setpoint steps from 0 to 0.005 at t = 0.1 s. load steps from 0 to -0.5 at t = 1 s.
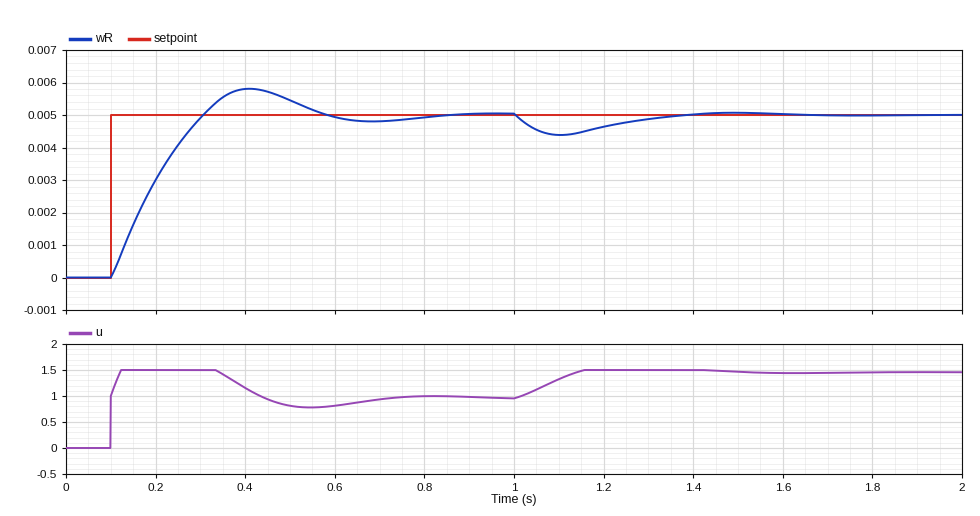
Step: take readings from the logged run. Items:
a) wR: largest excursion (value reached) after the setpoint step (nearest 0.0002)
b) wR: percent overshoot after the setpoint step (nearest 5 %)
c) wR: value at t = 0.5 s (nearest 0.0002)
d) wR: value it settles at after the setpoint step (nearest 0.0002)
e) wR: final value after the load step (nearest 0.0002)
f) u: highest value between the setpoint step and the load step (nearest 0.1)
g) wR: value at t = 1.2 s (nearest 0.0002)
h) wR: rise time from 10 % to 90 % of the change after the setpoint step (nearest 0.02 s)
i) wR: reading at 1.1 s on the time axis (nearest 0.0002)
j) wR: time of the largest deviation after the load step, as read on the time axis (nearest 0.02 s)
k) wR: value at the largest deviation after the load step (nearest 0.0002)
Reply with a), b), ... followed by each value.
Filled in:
a) 0.0058
b) 15 %
c) 0.0054
d) 0.0050
e) 0.0050
f) 1.5
g) 0.0046
h) 0.16 s
i) 0.0044
j) 1.10 s
k) 0.0044
